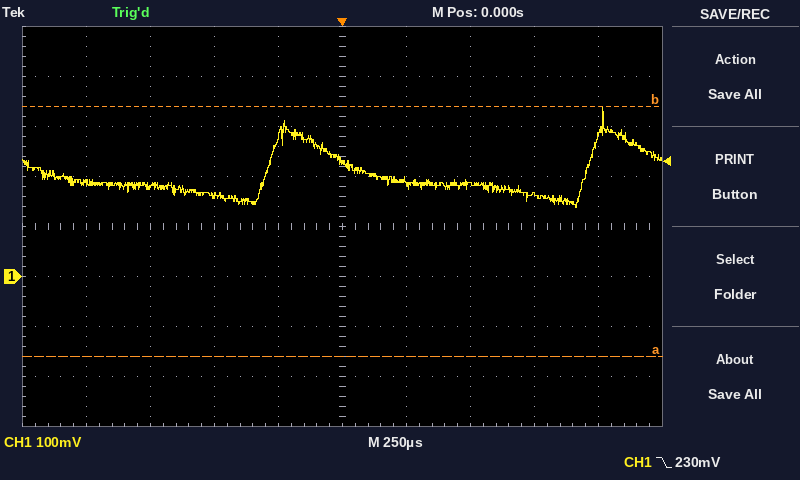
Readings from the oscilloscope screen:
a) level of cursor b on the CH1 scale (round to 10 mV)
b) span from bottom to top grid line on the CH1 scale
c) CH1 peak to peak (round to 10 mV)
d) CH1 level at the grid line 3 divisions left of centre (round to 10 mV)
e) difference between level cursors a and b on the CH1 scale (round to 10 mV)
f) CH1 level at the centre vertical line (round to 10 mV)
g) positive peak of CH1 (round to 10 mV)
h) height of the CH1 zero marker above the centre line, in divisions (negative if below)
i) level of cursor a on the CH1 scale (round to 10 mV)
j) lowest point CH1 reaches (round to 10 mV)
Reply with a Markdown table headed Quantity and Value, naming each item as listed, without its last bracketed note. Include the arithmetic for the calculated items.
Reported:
| Quantity | Value |
|---|---|
| level of cursor b on the CH1 scale | 340 mV |
| span from bottom to top grid line on the CH1 scale | 800 mV |
| CH1 peak to peak | 340 mV − (140 mV) = 200 mV |
| CH1 level at the grid line 3 divisions left of centre | 180 mV |
| difference between level cursors a and b on the CH1 scale | 500 mV |
| CH1 level at the centre vertical line | 230 mV |
| positive peak of CH1 | 340 mV |
| height of the CH1 zero marker above the centre line, in divisions | -1.0 div |
| level of cursor a on the CH1 scale | -160 mV |
| lowest point CH1 reaches | 140 mV |
